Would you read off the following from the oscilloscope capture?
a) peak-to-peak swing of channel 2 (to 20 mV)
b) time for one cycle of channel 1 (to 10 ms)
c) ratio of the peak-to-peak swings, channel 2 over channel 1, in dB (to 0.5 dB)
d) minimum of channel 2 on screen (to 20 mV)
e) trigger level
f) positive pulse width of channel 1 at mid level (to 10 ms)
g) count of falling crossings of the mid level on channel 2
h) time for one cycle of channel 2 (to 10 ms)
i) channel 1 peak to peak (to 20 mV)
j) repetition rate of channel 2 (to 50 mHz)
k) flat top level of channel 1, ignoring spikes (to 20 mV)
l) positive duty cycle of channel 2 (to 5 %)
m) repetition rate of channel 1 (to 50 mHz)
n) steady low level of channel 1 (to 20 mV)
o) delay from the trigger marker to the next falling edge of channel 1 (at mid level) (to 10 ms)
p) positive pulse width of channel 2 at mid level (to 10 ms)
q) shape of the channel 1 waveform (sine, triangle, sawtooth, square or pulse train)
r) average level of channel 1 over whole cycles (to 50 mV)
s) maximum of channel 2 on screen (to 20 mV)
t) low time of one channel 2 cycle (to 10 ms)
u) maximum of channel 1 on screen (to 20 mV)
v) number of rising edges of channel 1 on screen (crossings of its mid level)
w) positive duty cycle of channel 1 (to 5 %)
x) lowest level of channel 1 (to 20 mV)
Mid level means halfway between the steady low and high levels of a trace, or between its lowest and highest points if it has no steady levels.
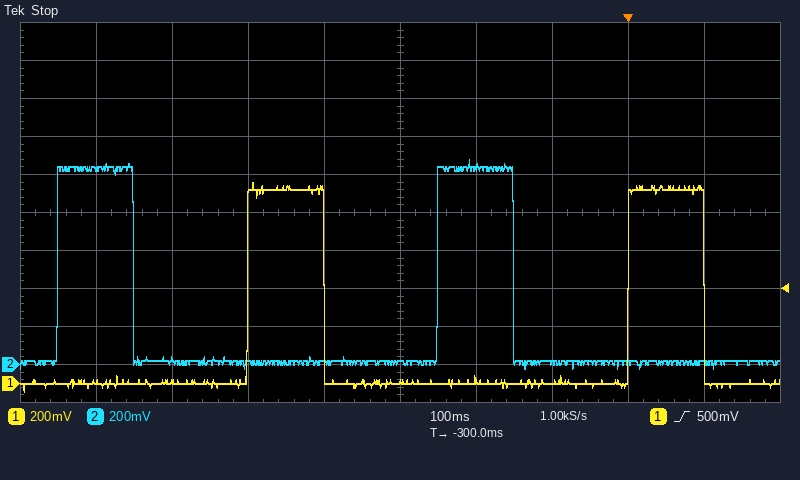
1.10 V
500 ms
0.0 dB
-20 mV
500 mV
100 ms
2
500 ms
1.10 V
2.00 Hz
1.02 V
20 %
2.00 Hz
0 mV
100 ms
100 ms
pulse train
200 mV
1.08 V
400 ms
1.06 V
2
20 %
-40 mV
